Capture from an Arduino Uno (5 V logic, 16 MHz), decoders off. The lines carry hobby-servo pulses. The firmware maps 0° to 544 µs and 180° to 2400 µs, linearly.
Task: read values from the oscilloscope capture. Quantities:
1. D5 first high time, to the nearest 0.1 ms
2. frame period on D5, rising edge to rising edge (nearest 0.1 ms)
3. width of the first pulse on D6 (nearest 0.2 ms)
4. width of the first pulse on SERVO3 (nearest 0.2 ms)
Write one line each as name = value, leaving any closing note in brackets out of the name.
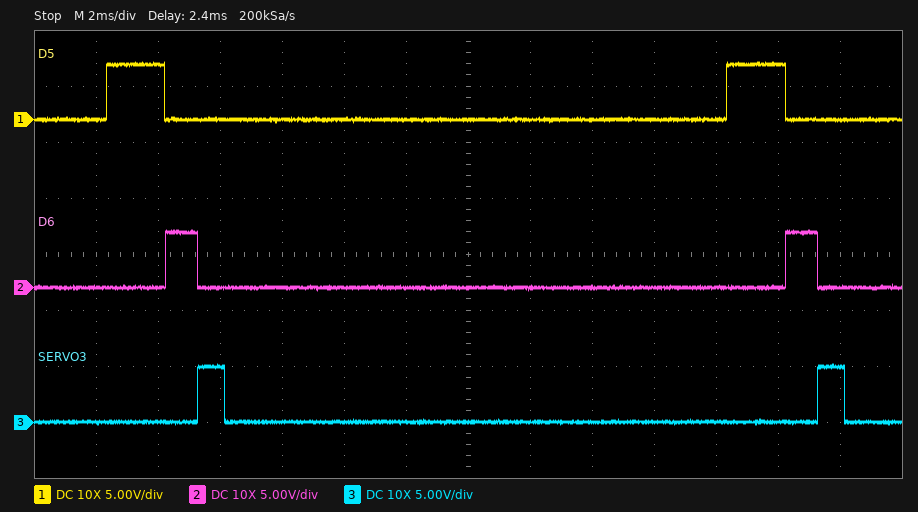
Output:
D5 first high time, to the nearest 0.1 ms = 1.9 ms
frame period on D5, rising edge to rising edge = 20.0 ms
width of the first pulse on D6 = 1.0 ms
width of the first pulse on SERVO3 = 0.8 ms
